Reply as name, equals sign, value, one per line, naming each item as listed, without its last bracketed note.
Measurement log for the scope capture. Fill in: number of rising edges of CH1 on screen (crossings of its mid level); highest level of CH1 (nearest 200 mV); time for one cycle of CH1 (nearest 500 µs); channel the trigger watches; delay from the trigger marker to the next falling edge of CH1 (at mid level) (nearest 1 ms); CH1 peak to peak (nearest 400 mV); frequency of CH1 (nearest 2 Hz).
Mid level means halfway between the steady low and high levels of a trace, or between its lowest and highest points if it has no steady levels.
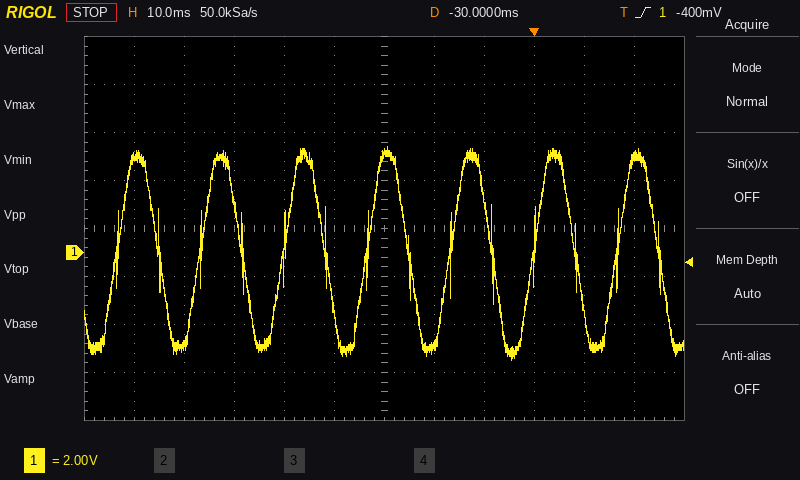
number of rising edges of CH1 on screen = 7
highest level of CH1 = 4.4 V
time for one cycle of CH1 = 16.5 ms
channel the trigger watches = CH1
delay from the trigger marker to the next falling edge of CH1 (at mid level) = 8 ms
CH1 peak to peak = 8.8 V
frequency of CH1 = 60 Hz
